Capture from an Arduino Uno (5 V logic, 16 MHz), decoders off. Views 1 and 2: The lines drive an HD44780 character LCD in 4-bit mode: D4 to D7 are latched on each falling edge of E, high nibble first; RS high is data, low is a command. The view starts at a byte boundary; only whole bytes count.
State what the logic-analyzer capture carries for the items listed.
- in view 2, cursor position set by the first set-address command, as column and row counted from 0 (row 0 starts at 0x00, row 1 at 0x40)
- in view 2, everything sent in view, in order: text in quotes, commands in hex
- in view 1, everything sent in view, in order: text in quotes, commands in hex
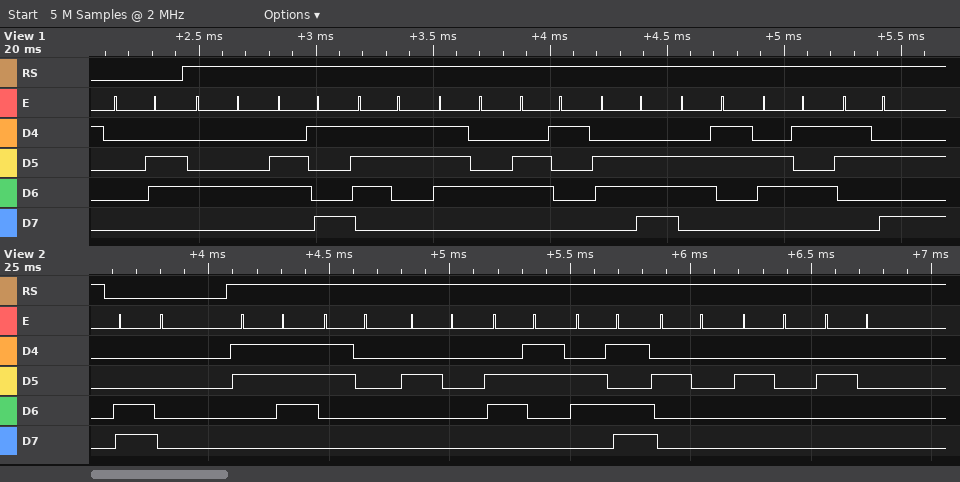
column 0, row 1
0xC0 "70 cm   "
0x06 "Distance:"
